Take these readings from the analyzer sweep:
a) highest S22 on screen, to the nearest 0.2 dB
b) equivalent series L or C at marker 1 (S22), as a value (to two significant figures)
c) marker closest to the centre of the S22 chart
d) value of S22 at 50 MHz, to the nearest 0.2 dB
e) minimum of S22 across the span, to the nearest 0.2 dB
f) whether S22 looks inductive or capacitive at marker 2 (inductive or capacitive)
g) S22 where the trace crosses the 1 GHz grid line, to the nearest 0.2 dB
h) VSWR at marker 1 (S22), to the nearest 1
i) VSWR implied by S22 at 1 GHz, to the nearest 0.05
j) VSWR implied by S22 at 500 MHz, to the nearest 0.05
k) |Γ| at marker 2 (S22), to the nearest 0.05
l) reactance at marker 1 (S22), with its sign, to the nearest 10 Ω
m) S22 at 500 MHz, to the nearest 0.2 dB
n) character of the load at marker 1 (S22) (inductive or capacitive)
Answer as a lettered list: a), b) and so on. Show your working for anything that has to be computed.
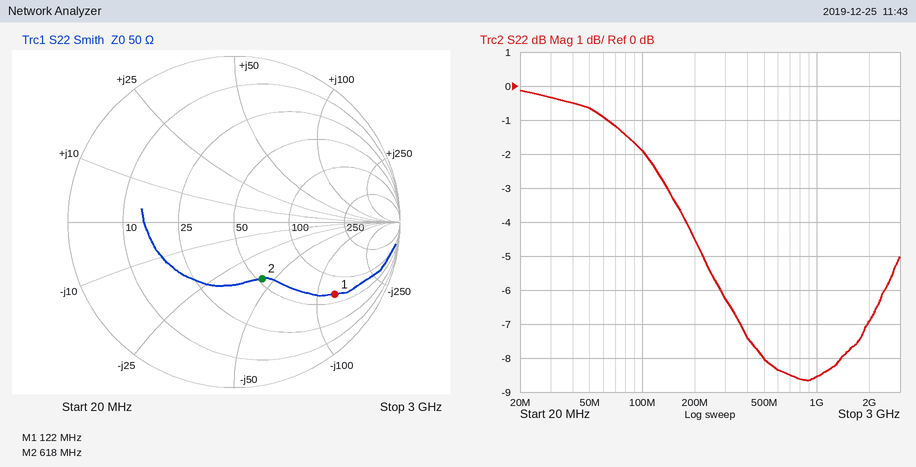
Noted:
a) -0.2 dB
b) C = 1/(2π × 122 MHz × 130 Ω) ≈ 10 pF
c) marker 2
d) -0.6 dB
e) -8.6 dB
f) capacitive
g) -8.6 dB
h) 7
i) |Γ| = 10^(-8.6/20) = 0.3715; VSWR = (1 + 0.3715)/(1 − 0.3715) ≈ 2.18, so 2.20 to the nearest 0.05
j) |Γ| = 10^(-8/20) = 0.3981; VSWR = (1 + 0.3981)/(1 − 0.3981) ≈ 2.32, so 2.30 to the nearest 0.05
k) 0.40
l) -130 Ω
m) -8.0 dB
n) capacitive
